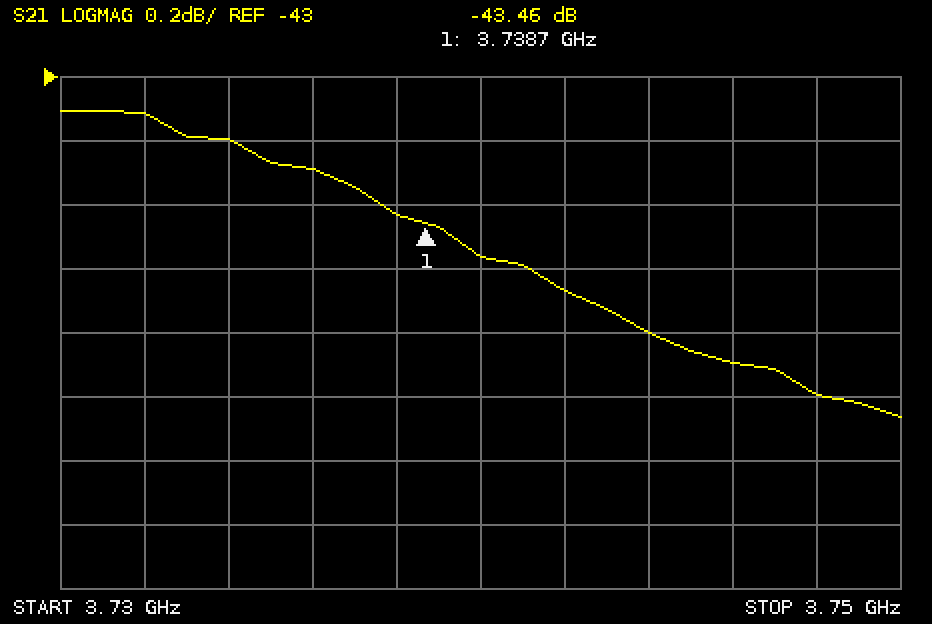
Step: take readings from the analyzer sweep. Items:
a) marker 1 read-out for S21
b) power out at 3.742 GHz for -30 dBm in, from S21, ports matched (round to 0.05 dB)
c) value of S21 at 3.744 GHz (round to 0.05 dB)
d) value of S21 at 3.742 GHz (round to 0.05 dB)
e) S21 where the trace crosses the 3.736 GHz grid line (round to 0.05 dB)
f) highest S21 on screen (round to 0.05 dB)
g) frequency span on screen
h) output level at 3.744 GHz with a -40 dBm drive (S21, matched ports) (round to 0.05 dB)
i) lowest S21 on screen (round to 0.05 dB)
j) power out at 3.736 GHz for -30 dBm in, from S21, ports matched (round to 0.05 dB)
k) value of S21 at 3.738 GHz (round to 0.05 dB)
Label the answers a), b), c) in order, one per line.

a) -43.46 dB
b) -73.65 dBm
c) -43.80 dB
d) -43.65 dB
e) -43.30 dB
f) -43.10 dB
g) 20 MHz
h) -83.80 dBm
i) -44.05 dB
j) -73.30 dBm
k) -43.45 dB
